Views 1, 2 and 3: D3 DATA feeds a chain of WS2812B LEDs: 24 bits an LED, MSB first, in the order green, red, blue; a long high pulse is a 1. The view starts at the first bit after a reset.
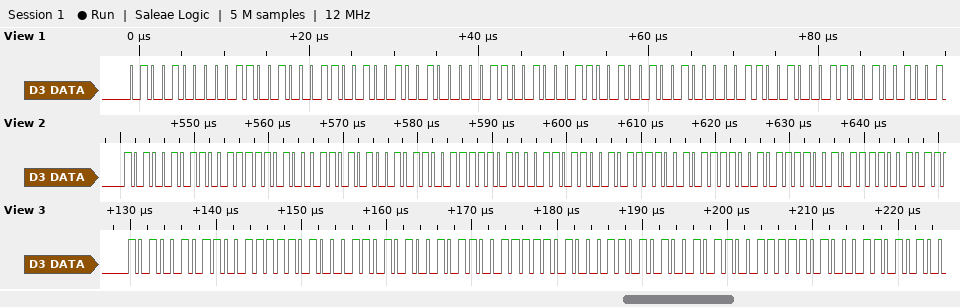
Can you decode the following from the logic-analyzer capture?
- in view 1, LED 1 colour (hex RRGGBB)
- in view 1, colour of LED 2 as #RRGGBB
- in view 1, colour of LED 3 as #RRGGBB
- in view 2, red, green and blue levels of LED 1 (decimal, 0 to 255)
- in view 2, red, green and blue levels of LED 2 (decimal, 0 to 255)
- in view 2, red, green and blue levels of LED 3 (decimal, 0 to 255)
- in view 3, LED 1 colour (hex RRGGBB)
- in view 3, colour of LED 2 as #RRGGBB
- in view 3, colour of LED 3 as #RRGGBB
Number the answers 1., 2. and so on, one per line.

1. #324832
2. #324832
3. #324832
4. 159, 165, 70
5. 159, 165, 70
6. 203, 203, 203
7. #9FA546
8. #9FA546
9. #9FA546
